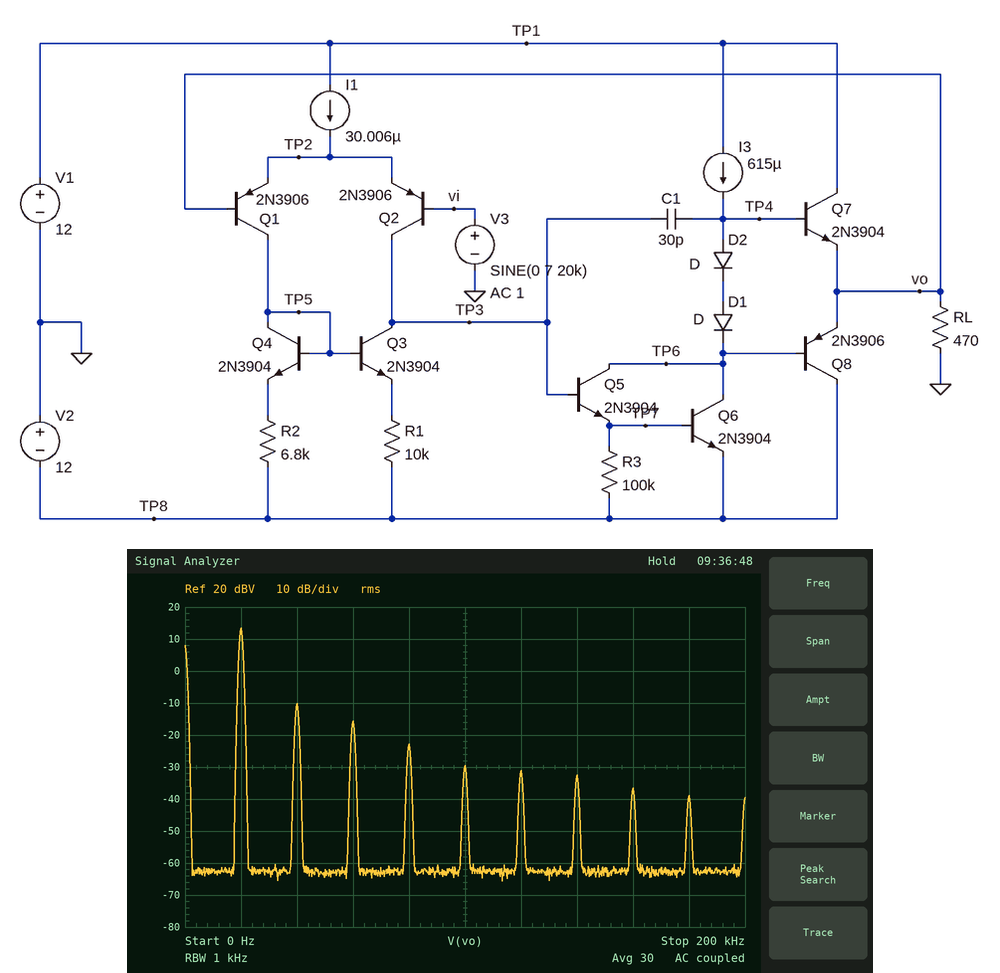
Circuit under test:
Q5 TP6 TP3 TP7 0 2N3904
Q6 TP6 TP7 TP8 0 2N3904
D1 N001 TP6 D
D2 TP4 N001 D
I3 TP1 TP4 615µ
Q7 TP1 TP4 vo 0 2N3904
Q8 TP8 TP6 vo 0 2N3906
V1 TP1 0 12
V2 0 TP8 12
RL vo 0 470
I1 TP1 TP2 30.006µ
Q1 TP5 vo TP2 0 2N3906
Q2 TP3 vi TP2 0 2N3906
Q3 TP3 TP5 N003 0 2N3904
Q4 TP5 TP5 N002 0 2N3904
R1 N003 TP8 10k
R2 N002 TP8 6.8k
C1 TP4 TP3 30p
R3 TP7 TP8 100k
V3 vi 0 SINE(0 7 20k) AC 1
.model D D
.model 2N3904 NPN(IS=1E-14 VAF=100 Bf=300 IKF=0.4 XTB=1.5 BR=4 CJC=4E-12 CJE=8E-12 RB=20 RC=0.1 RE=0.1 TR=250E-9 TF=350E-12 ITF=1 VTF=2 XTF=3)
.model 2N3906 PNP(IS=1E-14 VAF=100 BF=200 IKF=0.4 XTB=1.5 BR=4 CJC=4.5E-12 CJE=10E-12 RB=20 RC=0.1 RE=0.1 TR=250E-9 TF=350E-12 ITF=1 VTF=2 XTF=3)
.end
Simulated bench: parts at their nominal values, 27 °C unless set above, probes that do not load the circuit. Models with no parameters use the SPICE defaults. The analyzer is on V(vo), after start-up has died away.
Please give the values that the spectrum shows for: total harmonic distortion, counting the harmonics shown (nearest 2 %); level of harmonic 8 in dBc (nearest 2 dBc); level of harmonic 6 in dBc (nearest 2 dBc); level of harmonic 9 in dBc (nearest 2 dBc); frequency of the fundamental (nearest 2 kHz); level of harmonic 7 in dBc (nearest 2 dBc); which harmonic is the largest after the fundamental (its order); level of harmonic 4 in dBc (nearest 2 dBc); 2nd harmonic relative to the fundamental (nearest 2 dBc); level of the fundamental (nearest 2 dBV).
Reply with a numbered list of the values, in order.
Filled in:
1. 8 %
2. -50 dBc
3. -44 dBc
4. -52 dBc
5. 20 kHz
6. -46 dBc
7. 2
8. -36 dBc
9. -24 dBc
10. 14 dBV
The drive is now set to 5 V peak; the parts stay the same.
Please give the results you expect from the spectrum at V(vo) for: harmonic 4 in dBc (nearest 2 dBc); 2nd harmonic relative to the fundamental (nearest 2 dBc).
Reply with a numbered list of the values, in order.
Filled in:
1. -58 dBc
2. -52 dBc
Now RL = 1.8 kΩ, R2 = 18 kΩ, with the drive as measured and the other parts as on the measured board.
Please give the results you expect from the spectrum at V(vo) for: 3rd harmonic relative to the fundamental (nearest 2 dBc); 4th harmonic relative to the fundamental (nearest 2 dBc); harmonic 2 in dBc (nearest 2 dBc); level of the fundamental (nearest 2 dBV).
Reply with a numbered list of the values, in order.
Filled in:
1. -56 dBc
2. -60 dBc
3. -54 dBc
4. 14 dBV
